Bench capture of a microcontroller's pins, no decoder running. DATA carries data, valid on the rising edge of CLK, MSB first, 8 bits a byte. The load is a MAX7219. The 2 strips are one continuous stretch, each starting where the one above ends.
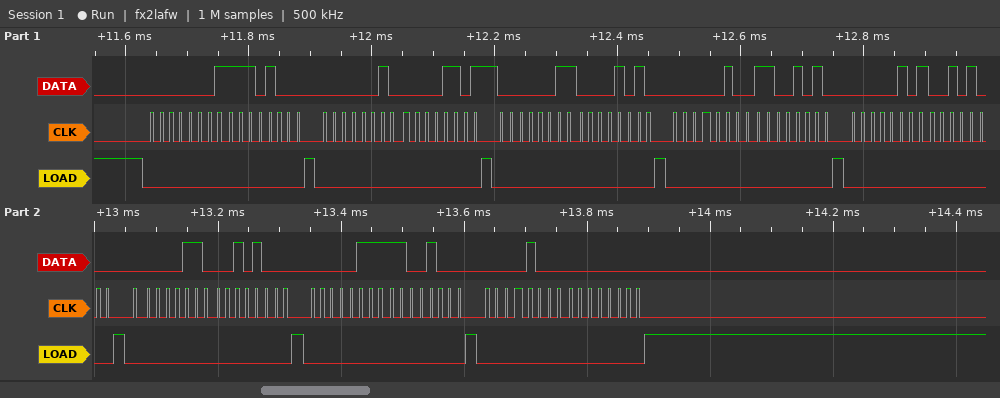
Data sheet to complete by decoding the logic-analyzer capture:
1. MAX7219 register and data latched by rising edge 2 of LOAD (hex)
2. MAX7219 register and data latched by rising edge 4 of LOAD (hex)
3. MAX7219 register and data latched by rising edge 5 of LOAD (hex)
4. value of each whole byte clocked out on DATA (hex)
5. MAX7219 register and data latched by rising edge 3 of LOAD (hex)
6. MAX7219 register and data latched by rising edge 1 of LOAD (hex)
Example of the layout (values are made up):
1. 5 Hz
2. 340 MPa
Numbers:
1. register 0x2, data 0x0D
2. register 0x4, data 0xCA
3. register 0x5, data 0x28
4. 01 E8 02 0D 03 0A 04 CA 05 28 06 28 07 C8 08 00
5. register 0x3, data 0x0A
6. register 0x1, data 0xE8
